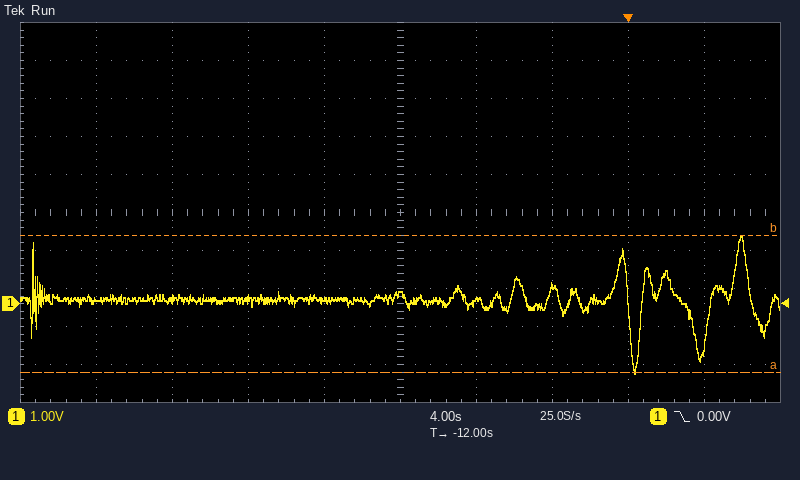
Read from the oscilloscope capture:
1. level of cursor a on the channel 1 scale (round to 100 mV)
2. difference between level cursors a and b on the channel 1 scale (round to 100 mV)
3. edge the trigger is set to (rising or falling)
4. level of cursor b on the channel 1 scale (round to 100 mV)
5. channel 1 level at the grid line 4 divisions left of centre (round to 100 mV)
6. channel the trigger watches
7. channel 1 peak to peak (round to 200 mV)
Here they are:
-1.8 V
3.6 V
falling
1.8 V
100 mV
channel 1
3.6 V
